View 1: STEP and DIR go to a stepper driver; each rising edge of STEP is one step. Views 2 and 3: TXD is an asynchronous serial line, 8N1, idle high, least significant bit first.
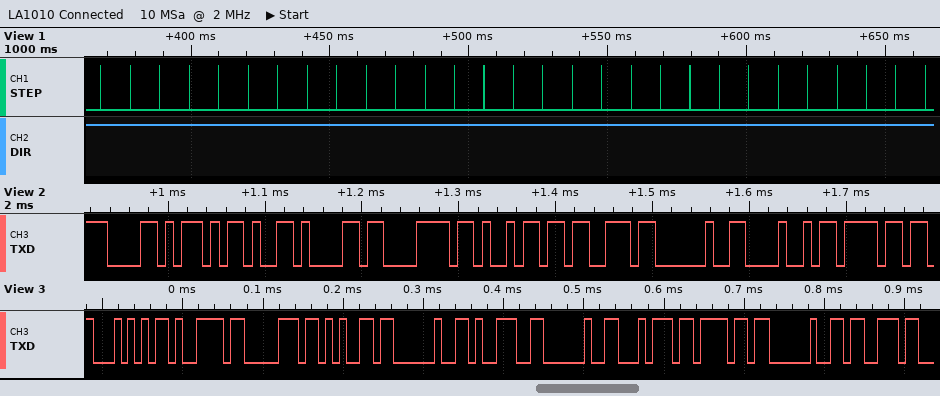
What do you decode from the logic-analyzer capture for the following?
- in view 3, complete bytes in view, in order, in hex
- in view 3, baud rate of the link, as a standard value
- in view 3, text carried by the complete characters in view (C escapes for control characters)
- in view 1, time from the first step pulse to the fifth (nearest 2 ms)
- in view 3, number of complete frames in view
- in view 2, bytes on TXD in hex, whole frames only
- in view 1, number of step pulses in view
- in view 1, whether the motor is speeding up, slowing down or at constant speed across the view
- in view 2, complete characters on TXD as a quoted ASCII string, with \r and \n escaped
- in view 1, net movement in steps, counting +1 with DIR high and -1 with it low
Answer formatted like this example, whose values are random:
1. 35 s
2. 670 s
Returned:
1. 54 79 70 65 20 39 20 74 6F 20 73
2. 115200 baud
3. "Type 9 to s"
4. 42 ms
5. 11
6. 58 2D 61 78 69 73 20 48 6F
7. 29
8. constant speed
9. "X-axis Ho"
10. +29
